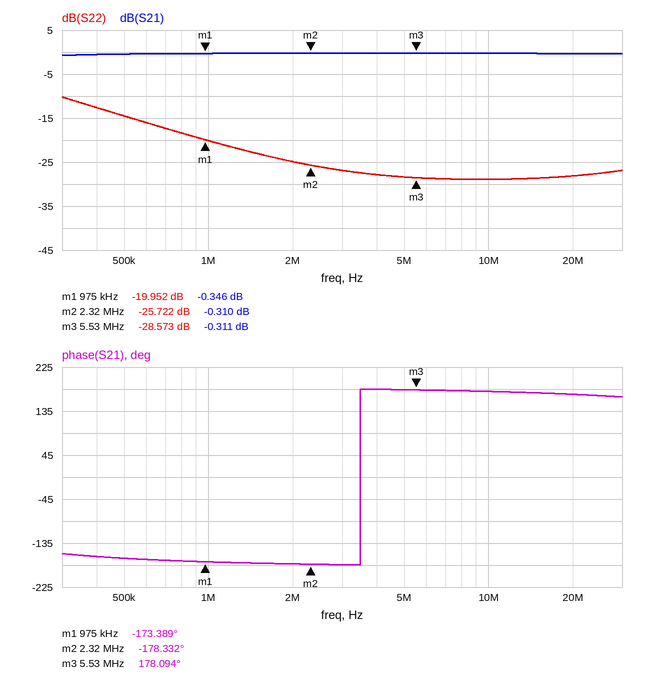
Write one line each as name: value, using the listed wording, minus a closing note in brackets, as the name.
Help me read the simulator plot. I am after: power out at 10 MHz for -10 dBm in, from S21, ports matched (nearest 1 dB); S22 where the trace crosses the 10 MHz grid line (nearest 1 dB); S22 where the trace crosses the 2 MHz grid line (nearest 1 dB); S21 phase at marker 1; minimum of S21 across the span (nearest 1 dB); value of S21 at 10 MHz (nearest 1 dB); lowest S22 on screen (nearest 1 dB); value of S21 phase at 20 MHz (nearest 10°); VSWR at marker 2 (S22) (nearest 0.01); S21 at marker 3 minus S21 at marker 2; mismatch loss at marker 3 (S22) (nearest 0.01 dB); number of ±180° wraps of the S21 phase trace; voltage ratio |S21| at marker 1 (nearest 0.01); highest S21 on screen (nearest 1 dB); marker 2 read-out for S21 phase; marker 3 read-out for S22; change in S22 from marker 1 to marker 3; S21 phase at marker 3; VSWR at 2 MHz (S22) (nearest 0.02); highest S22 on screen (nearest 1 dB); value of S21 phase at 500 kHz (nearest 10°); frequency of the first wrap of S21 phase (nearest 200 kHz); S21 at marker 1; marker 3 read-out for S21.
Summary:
power out at 10 MHz for -10 dBm in, from S21, ports matched: -10 dBm
S22 where the trace crosses the 10 MHz grid line: -29 dB
S22 where the trace crosses the 2 MHz grid line: -25 dB
S21 phase at marker 1: -173.389°
minimum of S21 across the span: -1 dB
value of S21 at 10 MHz: 0 dB
lowest S22 on screen: -29 dB
value of S21 phase at 20 MHz: 170°
VSWR at marker 2 (S22): 1.11
S21 at marker 3 minus S21 at marker 2: -0.001 dB
mismatch loss at marker 3 (S22): 0.01 dB
number of ±180° wraps of the S21 phase trace: 1
voltage ratio |S21| at marker 1: 0.96
highest S21 on screen: 0 dB
marker 2 read-out for S21 phase: -178.332°
marker 3 read-out for S22: -28.573 dB
change in S22 from marker 1 to marker 3: -8.621 dB
S21 phase at marker 3: 178.094°
VSWR at 2 MHz (S22): 1.12
highest S22 on screen: -10 dB
value of S21 phase at 500 kHz: -170°
frequency of the first wrap of S21 phase: 3.4 MHz
S21 at marker 1: -0.346 dB
marker 3 read-out for S21: -0.311 dB
